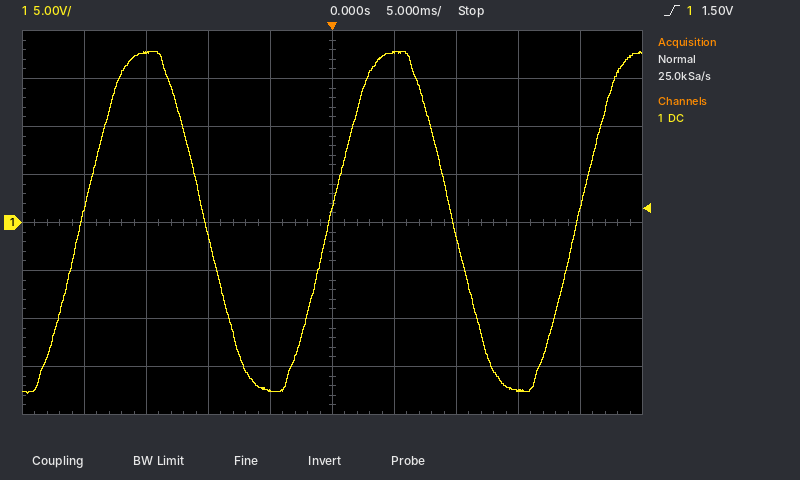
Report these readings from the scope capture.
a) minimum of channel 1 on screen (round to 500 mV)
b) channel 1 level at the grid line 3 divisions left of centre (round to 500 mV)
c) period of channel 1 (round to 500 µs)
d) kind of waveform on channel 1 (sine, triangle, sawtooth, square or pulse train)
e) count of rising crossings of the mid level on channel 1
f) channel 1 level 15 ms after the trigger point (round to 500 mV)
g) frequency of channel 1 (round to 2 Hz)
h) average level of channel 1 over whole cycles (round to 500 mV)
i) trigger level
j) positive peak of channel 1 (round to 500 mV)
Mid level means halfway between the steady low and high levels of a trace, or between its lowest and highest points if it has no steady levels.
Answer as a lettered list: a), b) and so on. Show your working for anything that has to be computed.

a) -18.0 V
b) 17.5 V
c) 20.0 ms
d) sine
e) 3
f) -17.5 V
g) 1 / 20.0 ms ≈ 50 Hz
h) (18.0 V + (-18.0 V)) / 2 ≈ 0.0 V
i) 1.50 V
j) 18.0 V
